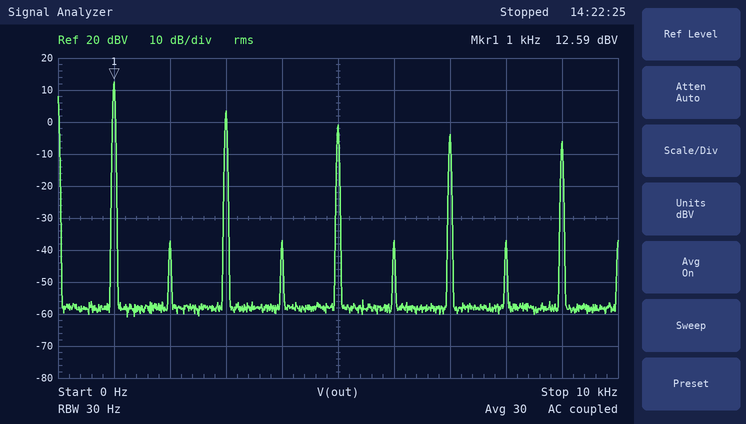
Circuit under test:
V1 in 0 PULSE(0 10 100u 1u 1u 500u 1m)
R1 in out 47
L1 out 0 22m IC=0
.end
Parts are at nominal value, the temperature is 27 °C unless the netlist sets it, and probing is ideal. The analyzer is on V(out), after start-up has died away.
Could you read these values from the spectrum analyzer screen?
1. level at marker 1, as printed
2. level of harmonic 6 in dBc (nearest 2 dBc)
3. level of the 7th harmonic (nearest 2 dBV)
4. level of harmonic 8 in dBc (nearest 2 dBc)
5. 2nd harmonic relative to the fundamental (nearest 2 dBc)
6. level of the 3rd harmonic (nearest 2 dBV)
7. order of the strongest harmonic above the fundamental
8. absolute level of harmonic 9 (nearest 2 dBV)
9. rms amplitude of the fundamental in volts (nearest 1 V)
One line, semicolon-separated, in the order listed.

12.59 dBV; -50 dBc; -4 dBV; -50 dBc; -50 dBc; 4 dBV; 3; -6 dBV; 4 V
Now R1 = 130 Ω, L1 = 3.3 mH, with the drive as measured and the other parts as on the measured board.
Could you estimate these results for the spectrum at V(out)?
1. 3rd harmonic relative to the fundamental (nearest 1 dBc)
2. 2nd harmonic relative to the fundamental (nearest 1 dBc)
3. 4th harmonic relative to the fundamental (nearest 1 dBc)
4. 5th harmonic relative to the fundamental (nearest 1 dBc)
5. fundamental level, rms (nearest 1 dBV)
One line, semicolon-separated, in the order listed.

-1 dBc; -44 dBc; -39 dBc; -2 dBc; -3 dBV
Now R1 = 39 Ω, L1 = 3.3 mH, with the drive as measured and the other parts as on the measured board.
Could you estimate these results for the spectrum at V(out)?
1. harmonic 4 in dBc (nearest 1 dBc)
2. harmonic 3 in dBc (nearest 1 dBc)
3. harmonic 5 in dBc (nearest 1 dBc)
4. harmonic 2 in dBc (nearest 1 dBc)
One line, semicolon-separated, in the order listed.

-44 dBc; -4 dBc; -8 dBc; -46 dBc
